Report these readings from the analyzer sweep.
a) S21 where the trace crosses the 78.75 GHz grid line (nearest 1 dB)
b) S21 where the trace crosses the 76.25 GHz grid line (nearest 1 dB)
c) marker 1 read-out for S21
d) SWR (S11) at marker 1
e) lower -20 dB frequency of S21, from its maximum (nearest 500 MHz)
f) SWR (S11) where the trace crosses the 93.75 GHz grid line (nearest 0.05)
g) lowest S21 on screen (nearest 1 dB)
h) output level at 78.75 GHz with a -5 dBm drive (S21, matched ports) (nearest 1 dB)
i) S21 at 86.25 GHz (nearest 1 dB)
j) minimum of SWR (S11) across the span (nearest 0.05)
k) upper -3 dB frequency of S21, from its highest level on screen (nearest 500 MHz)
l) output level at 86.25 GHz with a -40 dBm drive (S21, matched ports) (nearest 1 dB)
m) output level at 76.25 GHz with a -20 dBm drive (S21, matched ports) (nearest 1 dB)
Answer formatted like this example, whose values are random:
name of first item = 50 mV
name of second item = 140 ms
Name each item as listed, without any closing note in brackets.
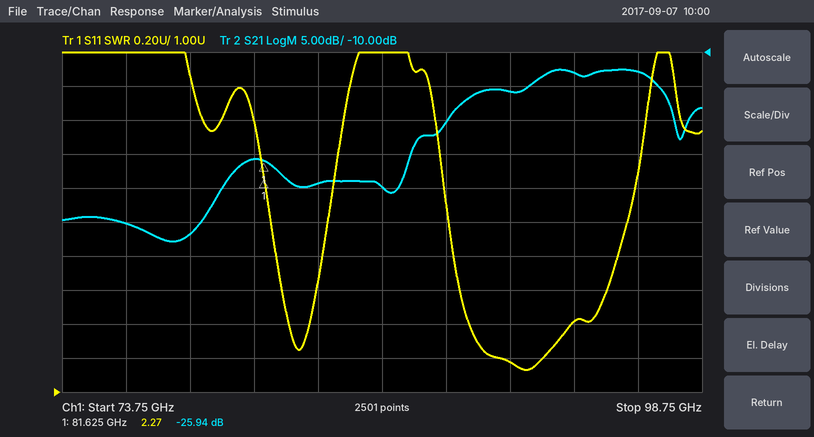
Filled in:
S21 where the trace crosses the 78.75 GHz grid line = -37 dB
S21 where the trace crosses the 76.25 GHz grid line = -35 dB
marker 1 read-out for S21 = -25.94 dB
SWR (S11) at marker 1 = 2.27
lower -20 dB frequency of S21, from its maximum = 79.5 GHz
SWR (S11) where the trace crosses the 93.75 GHz grid line = 1.40
lowest S21 on screen = -38 dB
output level at 78.75 GHz with a -5 dBm drive (S21, matched ports) = -42 dBm
S21 at 86.25 GHz = -30 dB
minimum of SWR (S11) across the span = 1.15
upper -3 dB frequency of S21, from its highest level on screen = 97.0 GHz
output level at 86.25 GHz with a -40 dBm drive (S21, matched ports) = -70 dBm
output level at 76.25 GHz with a -20 dBm drive (S21, matched ports) = -55 dBm
